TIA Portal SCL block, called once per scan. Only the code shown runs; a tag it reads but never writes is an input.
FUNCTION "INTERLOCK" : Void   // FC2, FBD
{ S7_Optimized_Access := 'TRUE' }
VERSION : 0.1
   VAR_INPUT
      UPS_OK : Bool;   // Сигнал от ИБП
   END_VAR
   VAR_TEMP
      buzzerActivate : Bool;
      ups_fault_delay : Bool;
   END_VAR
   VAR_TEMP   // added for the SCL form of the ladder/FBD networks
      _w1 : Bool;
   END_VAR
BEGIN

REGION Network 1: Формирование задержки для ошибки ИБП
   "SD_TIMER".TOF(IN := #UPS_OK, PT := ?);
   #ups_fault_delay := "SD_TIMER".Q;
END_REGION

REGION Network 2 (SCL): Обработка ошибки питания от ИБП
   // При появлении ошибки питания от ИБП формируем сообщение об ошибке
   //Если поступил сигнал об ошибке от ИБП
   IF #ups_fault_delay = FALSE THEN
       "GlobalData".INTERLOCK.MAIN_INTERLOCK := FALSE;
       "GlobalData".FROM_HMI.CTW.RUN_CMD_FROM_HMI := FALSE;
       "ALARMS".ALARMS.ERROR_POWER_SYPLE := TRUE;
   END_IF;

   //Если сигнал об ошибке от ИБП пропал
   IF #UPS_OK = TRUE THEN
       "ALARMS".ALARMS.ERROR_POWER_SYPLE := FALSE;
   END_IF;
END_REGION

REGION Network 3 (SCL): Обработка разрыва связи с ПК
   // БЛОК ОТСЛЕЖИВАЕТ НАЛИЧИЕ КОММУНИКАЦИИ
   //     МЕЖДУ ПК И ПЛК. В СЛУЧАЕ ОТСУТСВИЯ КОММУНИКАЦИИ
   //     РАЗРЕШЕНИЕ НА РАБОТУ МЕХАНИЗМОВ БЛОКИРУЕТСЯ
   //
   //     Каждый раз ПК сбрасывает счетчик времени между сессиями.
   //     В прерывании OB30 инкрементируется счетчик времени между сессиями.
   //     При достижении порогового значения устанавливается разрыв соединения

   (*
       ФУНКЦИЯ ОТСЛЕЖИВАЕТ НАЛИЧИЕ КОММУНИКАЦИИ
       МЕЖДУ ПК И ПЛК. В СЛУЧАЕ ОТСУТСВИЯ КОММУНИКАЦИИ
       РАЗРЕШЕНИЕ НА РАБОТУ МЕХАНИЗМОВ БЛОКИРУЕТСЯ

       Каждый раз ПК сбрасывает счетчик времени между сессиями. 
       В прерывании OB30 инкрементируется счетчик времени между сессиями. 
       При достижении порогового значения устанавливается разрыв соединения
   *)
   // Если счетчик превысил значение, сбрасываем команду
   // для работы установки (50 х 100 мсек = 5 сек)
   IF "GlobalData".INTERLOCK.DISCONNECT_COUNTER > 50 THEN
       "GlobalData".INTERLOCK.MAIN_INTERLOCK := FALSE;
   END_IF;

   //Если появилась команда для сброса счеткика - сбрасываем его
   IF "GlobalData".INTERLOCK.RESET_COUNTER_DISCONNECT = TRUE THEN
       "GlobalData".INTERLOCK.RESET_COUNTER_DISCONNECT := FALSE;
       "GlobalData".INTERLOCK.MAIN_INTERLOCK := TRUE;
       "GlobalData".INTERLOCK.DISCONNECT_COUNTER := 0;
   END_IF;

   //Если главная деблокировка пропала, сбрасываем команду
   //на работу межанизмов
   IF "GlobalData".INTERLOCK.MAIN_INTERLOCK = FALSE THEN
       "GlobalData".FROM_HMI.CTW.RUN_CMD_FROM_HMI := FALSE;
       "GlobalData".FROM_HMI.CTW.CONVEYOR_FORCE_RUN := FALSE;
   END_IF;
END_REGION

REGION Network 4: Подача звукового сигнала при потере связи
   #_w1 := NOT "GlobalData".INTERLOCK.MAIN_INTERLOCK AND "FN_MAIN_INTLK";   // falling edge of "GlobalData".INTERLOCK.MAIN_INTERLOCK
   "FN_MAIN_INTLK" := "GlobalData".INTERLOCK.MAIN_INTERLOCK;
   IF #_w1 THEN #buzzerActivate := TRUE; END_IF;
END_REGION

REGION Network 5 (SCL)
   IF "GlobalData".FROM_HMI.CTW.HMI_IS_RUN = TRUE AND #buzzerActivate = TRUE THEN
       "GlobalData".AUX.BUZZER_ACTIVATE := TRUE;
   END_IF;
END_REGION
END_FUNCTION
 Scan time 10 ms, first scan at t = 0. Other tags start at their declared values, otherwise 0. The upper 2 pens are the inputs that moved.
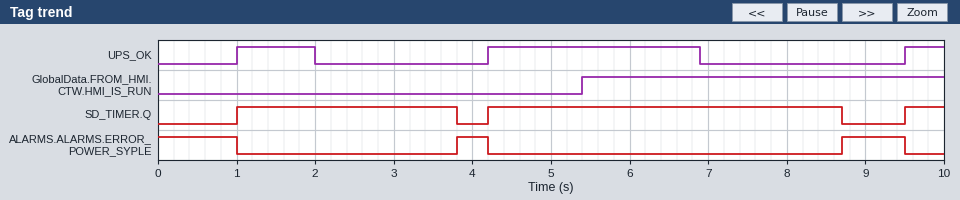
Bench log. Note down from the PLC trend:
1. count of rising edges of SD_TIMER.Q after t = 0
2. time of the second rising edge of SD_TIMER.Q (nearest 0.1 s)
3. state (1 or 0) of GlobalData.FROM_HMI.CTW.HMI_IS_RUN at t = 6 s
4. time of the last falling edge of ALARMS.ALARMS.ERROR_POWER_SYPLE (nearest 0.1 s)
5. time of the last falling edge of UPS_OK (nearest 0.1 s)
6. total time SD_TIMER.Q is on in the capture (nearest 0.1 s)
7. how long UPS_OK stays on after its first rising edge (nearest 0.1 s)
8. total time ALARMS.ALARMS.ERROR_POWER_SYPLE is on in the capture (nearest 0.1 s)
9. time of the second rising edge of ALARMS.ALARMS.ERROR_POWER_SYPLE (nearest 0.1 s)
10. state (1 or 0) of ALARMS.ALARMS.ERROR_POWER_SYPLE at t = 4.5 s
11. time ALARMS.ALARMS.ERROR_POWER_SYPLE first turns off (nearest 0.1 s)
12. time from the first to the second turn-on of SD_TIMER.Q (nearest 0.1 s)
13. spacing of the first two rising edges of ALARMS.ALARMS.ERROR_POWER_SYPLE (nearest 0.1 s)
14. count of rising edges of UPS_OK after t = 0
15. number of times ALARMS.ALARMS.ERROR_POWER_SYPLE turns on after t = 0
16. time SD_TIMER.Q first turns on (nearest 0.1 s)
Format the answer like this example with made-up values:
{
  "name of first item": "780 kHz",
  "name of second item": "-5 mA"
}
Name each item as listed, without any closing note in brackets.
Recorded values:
{
  "count of rising edges of SD_TIMER.Q after t = 0": "3",
  "time of the second rising edge of SD_TIMER.Q": "4.2 s",
  "state (1 or 0) of GlobalData.FROM_HMI.CTW.HMI_IS_RUN at t = 6 s": "1",
  "time of the last falling edge of ALARMS.ALARMS.ERROR_POWER_SYPLE": "9.5 s",
  "time of the last falling edge of UPS_OK": "6.9 s",
  "total time SD_TIMER.Q is on in the capture": "7.8 s",
  "how long UPS_OK stays on after its first rising edge": "1.0 s",
  "total time ALARMS.ALARMS.ERROR_POWER_SYPLE is on in the capture": "2.2 s",
  "time of the second rising edge of ALARMS.ALARMS.ERROR_POWER_SYPLE": "8.7 s",
  "state (1 or 0) of ALARMS.ALARMS.ERROR_POWER_SYPLE at t = 4.5 s": "0",
  "time ALARMS.ALARMS.ERROR_POWER_SYPLE first turns off": "1.0 s",
  "time from the first to the second turn-on of SD_TIMER.Q": "3.2 s",
  "spacing of the first two rising edges of ALARMS.ALARMS.ERROR_POWER_SYPLE": "4.9 s",
  "count of rising edges of UPS_OK after t = 0": "3",
  "number of times ALARMS.ALARMS.ERROR_POWER_SYPLE turns on after t = 0": "2",
  "time SD_TIMER.Q first turns on": "1.0 s"
}
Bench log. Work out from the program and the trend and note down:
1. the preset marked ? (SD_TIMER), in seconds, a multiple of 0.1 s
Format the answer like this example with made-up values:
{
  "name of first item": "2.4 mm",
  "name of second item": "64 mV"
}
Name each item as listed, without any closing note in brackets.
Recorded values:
{
  "the preset marked ? (SD_TIMER), in seconds, a multiple of 0.1 s": "1.8 s"
}
